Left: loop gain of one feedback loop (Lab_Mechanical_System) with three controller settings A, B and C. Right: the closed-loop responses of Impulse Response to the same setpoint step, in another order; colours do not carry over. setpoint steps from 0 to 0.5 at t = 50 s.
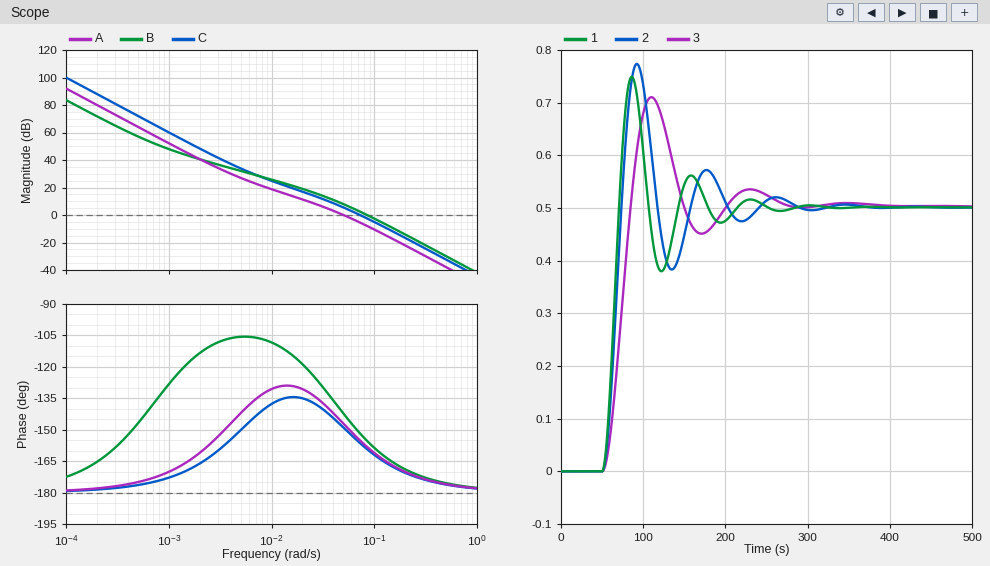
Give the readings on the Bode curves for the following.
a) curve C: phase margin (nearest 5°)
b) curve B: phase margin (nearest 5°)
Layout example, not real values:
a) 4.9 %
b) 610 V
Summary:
a) 25°
b) 25°
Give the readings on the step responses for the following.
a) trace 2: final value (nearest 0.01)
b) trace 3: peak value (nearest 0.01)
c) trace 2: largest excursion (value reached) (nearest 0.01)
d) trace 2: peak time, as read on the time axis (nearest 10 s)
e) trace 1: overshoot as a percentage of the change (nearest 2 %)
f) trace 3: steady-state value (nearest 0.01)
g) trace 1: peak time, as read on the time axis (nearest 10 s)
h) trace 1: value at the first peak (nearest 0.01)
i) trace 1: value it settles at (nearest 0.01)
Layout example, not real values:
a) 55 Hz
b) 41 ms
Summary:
a) 0.50
b) 0.71
c) 0.77
d) 90 s
e) 50 %
f) 0.50
g) 90 s
h) 0.75
i) 0.50
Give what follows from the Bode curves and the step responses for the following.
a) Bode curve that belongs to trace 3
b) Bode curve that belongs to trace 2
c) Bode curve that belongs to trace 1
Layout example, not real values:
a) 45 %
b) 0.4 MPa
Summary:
a) A
b) C
c) B
